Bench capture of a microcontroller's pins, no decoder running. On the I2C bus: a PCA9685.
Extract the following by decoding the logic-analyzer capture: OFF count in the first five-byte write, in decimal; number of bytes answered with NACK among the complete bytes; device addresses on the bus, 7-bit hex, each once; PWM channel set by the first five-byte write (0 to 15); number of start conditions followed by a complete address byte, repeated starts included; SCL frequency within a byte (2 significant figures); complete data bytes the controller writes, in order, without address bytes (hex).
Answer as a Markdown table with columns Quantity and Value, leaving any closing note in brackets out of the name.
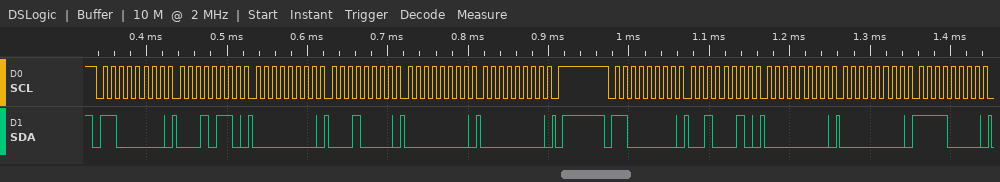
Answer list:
| Quantity | Value |
|---|---|
| OFF count in the first five-byte write, in decimal | 0 |
| number of bytes answered with NACK among the complete bytes | 0 |
| device addresses on the bus, 7-bit hex, each once | 0x60 |
| PWM channel set by the first five-byte write | 4 |
| number of start conditions followed by a complete address byte, repeated starts included | 2 |
| SCL frequency within a byte | 100 kHz |
| complete data bytes the controller writes, in order, without address bytes | 16 00 10 00 00 22 00 00 F0 |
